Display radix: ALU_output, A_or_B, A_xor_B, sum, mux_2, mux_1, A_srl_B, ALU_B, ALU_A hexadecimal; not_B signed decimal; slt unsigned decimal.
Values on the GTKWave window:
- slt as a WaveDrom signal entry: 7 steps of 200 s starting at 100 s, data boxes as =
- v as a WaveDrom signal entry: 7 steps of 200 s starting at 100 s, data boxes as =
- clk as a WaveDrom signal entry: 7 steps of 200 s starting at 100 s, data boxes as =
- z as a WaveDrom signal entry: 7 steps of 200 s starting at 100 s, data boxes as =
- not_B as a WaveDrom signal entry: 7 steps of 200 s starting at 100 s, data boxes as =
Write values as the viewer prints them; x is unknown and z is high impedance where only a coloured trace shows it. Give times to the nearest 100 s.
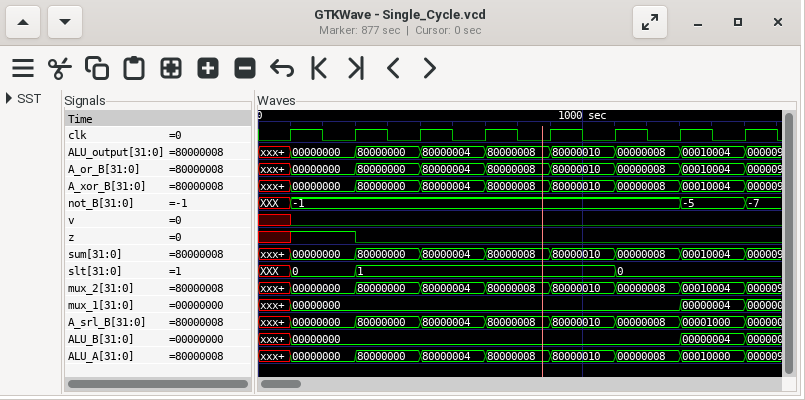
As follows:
{name: 'slt', wave: '==...=.', data: '0 1 0'}
{name: 'v', wave: '0......'}
{name: 'clk', wave: 'p......'}
{name: 'z', wave: '10.....'}
{name: 'not_B', wave: '=.....=', data: '-1 -5'}
